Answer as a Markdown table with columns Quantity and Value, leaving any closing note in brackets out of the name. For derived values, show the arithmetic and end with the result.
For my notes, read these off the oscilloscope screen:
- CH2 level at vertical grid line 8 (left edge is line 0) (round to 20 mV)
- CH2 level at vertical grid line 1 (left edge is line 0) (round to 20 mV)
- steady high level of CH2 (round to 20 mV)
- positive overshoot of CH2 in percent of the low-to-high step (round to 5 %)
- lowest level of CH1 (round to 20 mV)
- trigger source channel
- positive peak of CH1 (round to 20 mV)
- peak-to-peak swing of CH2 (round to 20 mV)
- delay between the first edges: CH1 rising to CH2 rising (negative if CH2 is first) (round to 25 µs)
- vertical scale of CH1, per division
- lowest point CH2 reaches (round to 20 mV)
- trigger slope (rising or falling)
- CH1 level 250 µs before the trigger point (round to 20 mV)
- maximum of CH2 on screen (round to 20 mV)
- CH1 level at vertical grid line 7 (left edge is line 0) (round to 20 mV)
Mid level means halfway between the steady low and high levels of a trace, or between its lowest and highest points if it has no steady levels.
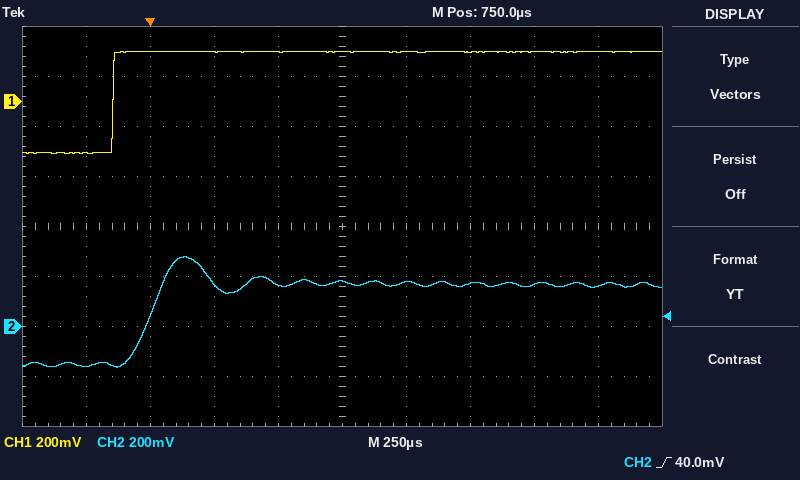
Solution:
| Quantity | Value |
|---|---|
| CH2 level at vertical grid line 8 (left edge is line 0) | 160 mV |
| CH2 level at vertical grid line 1 (left edge is line 0) | -160 mV |
| steady high level of CH2 | 160 mV |
| positive overshoot of CH2 in percent of the low-to-high step | 35 % |
| lowest level of CH1 | -200 mV |
| trigger source channel | CH2 |
| positive peak of CH1 | 200 mV |
| peak-to-peak swing of CH2 | 280 mV − (-160 mV) = 440 mV |
| delay between the first edges: CH1 rising to CH2 rising (negative if CH2 is first) | +125 µs |
| vertical scale of CH1, per division | 200 mV |
| lowest point CH2 reaches | -160 mV |
| trigger slope | rising |
| CH1 level 250 µs before the trigger point | -200 mV |
| maximum of CH2 on screen | 280 mV |
| CH1 level at vertical grid line 7 (left edge is line 0) | 200 mV |
